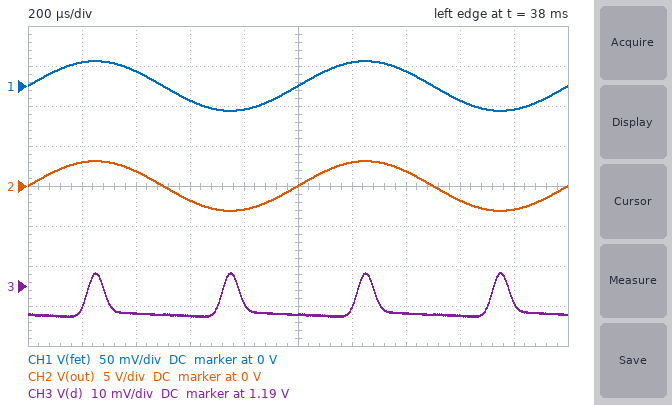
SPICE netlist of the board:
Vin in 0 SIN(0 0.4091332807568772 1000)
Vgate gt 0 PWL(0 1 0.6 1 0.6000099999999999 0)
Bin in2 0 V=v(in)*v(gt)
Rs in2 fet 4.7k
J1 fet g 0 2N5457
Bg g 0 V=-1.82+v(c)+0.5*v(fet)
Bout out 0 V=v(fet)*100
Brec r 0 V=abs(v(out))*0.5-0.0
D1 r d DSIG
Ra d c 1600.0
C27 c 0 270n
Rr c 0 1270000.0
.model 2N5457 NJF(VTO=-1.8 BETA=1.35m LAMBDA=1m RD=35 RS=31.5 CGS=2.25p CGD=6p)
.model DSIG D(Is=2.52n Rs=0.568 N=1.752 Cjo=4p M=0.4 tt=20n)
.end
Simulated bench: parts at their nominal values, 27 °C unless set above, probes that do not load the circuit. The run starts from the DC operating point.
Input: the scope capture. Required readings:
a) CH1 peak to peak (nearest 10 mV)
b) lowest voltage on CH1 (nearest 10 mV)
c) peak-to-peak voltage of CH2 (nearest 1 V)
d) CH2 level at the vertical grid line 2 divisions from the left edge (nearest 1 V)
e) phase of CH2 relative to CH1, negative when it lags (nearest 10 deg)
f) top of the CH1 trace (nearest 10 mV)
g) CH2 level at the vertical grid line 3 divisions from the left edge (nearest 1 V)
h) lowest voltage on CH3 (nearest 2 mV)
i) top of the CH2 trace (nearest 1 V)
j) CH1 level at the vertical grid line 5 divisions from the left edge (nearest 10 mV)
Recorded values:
60 mV
-30 mV
6 V
2 V
0 deg
30 mV
-2 V
1.182 V
3 V
0 V
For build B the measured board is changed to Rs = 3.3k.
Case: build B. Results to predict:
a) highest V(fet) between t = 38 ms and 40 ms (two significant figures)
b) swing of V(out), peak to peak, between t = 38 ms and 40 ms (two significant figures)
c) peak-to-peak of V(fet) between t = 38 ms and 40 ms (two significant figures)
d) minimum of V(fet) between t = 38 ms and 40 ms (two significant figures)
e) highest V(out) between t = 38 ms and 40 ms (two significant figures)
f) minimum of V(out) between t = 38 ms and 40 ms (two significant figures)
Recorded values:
37 mV
7.3 V
73 mV
-37 mV
3.7 V
-3.7 V
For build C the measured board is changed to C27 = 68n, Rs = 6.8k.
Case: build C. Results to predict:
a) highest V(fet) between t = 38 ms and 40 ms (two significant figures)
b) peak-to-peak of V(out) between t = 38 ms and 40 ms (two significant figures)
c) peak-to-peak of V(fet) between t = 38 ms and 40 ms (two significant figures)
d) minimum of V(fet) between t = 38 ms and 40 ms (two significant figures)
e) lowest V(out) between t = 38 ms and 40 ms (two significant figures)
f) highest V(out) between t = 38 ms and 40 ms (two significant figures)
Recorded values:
26 mV
5.2 V
52 mV
-26 mV
-2.6 V
2.6 V
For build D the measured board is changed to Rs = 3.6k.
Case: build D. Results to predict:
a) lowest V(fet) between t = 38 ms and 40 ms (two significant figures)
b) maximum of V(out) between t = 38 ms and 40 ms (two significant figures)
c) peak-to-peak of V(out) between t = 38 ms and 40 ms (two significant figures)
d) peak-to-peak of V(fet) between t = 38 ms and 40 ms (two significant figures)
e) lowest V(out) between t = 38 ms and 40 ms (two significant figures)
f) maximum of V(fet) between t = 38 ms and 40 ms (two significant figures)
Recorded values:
-35 mV
3.5 V
7.0 V
70 mV
-3.5 V
35 mV
